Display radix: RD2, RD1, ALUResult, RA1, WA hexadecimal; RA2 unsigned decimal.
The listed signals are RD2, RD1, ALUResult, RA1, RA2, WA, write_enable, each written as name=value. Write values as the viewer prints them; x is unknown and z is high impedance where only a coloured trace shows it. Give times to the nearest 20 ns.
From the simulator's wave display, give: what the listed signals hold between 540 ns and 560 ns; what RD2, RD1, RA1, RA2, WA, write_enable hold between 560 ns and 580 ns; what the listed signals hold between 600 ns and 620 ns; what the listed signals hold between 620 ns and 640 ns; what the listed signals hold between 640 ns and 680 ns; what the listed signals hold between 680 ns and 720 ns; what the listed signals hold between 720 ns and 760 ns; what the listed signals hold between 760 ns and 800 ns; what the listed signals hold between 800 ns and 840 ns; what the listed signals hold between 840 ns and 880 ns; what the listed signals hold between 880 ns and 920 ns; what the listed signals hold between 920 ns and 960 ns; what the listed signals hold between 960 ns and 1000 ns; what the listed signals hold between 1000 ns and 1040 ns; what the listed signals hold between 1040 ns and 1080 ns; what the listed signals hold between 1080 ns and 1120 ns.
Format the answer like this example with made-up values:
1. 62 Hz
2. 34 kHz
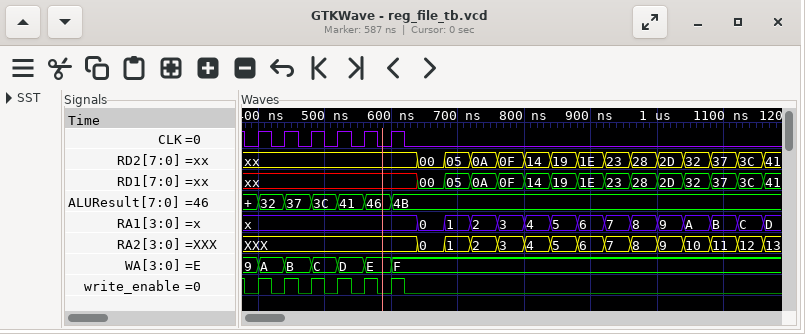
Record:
1. RD2=xx, RD1=xx, ALUResult=41, RA1=x, RA2=XXX, WA=D, write_enable=0
2. RD2=xx, RD1=xx, RA1=x, RA2=XXX, WA=E, write_enable=1
3. RD2=xx, RD1=xx, ALUResult=4B, RA1=x, RA2=XXX, WA=F, write_enable=1
4. RD2=xx, RD1=xx, ALUResult=4B, RA1=x, RA2=XXX, WA=F, write_enable=0
5. RD2=00, RD1=00, ALUResult=4B, RA1=0, RA2=0, WA=F, write_enable=0
6. RD2=05, RD1=05, ALUResult=4B, RA1=1, RA2=1, WA=F, write_enable=0
7. RD2=0A, RD1=0A, ALUResult=4B, RA1=2, RA2=2, WA=F, write_enable=0
8. RD2=0F, RD1=0F, ALUResult=4B, RA1=3, RA2=3, WA=F, write_enable=0
9. RD2=14, RD1=14, ALUResult=4B, RA1=4, RA2=4, WA=F, write_enable=0
10. RD2=19, RD1=19, ALUResult=4B, RA1=5, RA2=5, WA=F, write_enable=0
11. RD2=1E, RD1=1E, ALUResult=4B, RA1=6, RA2=6, WA=F, write_enable=0
12. RD2=23, RD1=23, ALUResult=4B, RA1=7, RA2=7, WA=F, write_enable=0
13. RD2=28, RD1=28, ALUResult=4B, RA1=8, RA2=8, WA=F, write_enable=0
14. RD2=2D, RD1=2D, ALUResult=4B, RA1=9, RA2=9, WA=F, write_enable=0
15. RD2=32, RD1=32, ALUResult=4B, RA1=A, RA2=10, WA=F, write_enable=0
16. RD2=37, RD1=37, ALUResult=4B, RA1=B, RA2=11, WA=F, write_enable=0
